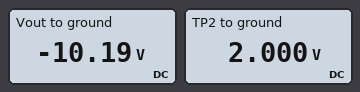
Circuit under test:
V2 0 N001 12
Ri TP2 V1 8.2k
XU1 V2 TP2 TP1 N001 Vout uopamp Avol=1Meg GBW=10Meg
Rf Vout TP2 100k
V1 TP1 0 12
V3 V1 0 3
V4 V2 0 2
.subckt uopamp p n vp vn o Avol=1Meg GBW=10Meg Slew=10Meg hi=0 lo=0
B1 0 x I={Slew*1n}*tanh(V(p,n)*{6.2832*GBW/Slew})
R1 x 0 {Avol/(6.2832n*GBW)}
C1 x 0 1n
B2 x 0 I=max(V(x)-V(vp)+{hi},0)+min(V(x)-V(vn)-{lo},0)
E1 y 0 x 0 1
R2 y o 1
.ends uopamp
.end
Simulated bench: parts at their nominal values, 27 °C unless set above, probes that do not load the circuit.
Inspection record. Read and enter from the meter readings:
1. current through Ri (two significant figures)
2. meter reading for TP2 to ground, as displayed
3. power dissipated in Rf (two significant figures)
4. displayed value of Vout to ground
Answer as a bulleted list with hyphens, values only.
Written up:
- 120 µA
- 2.000 V
- 1.5 mW
- -10.19 V
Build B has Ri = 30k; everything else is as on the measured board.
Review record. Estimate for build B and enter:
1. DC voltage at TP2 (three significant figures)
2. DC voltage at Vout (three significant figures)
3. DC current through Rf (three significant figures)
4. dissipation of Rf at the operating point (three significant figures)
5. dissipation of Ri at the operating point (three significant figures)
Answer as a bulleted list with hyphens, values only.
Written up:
- 2.00 V
- -1.33 V
- 33.3 µA
- 111 µW
- 33.3 µW
